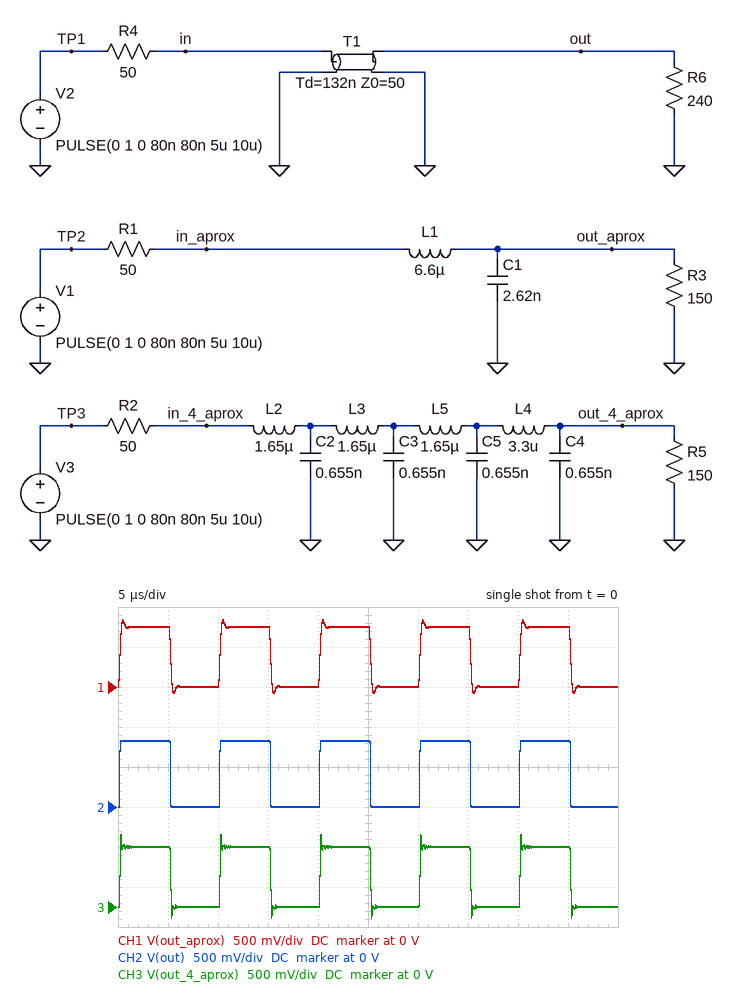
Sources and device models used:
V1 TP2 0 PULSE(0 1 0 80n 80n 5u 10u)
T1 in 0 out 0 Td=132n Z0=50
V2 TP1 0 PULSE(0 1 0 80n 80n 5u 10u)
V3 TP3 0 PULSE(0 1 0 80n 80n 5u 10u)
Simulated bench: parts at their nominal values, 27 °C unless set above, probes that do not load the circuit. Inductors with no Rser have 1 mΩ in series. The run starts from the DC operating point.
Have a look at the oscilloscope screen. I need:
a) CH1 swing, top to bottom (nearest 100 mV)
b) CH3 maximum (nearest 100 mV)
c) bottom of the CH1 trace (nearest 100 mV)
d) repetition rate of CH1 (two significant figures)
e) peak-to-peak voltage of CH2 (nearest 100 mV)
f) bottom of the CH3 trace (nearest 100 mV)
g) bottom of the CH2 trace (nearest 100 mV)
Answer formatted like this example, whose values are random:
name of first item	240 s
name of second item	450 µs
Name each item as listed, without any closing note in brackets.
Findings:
CH1 swing, top to bottom	900 mV
CH3 maximum	900 mV
bottom of the CH1 trace	-100 mV
repetition rate of CH1	100 kHz
peak-to-peak voltage of CH2	800 mV
bottom of the CH3 trace	-100 mV
bottom of the CH2 trace	0 V
